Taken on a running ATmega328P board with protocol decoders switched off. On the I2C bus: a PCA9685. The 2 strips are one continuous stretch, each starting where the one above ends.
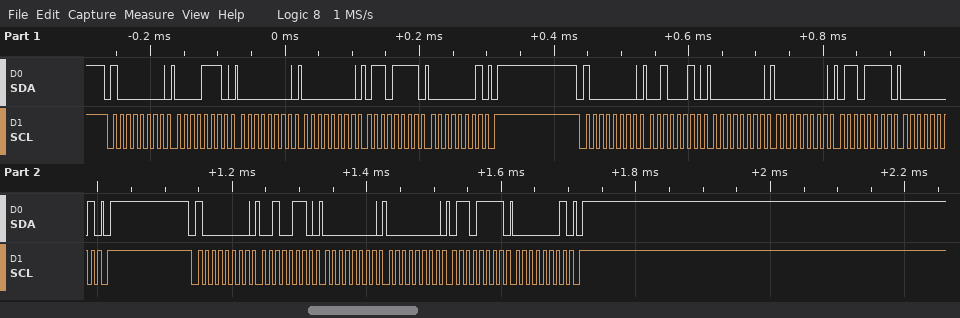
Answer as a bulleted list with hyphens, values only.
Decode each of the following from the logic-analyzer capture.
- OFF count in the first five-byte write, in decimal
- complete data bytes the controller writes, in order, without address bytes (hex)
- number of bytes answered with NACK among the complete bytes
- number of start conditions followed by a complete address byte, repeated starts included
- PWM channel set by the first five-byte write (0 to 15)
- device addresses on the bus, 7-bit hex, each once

- 367
- 0E 00 00 6F 01 22 00 00 6F 01 26 00 00 6F 01
- 0
- 3
- 2
- 0x40
